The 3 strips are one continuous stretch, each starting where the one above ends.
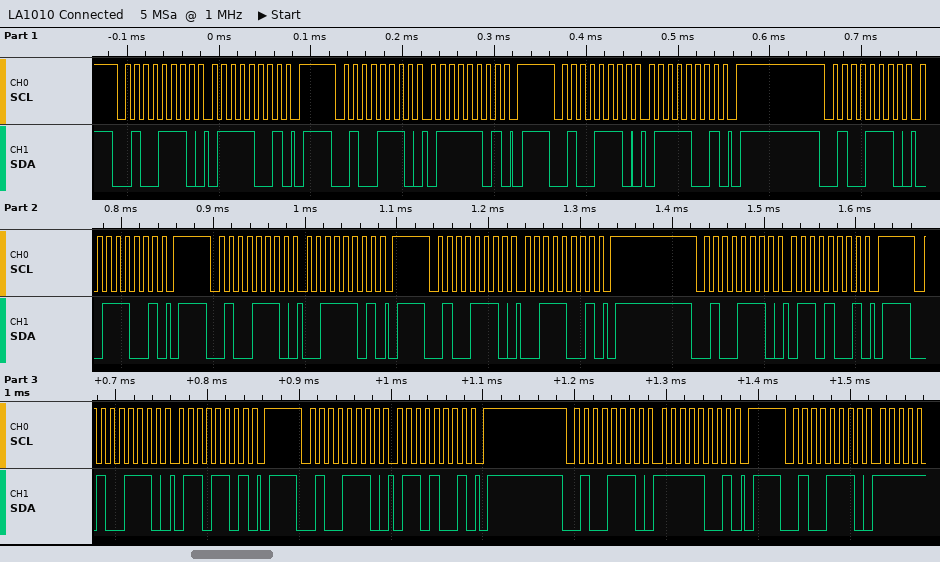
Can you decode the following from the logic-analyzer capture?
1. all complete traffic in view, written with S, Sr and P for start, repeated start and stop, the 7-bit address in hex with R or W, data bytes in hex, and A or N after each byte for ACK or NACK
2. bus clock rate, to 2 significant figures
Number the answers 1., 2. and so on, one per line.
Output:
1. S 27W A 79 A P S 27W A 7D A P S 27W A 79 A P S 27W A 39 A P S 27W A 3D A P S 27W A 39 A P S 27W A 69 A P S 27W A 6D A P S 27W A 69 A P S 27W A F9 A P S 27W A
2. 100 kHz
